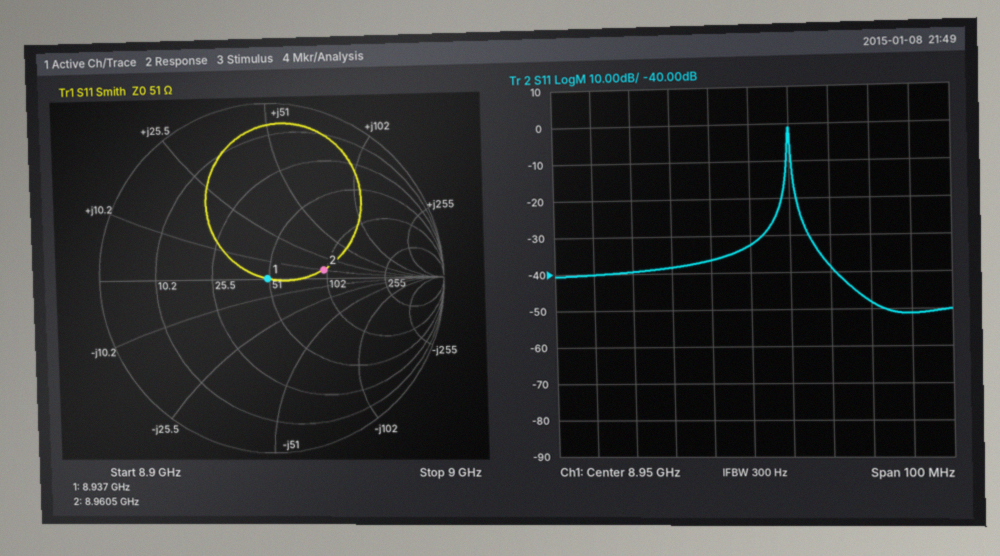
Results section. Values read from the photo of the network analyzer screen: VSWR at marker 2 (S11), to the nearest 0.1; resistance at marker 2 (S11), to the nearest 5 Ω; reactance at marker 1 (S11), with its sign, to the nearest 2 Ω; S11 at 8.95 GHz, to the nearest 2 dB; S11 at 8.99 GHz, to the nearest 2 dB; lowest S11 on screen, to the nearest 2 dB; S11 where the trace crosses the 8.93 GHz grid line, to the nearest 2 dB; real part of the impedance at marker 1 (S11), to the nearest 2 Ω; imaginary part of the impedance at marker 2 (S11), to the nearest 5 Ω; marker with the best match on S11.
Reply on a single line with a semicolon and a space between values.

1.9; 95 Ω; 0 Ω; -32 dB; -52 dB; -52 dB; -38 dB; 50 Ω; +10 Ω; marker 1
